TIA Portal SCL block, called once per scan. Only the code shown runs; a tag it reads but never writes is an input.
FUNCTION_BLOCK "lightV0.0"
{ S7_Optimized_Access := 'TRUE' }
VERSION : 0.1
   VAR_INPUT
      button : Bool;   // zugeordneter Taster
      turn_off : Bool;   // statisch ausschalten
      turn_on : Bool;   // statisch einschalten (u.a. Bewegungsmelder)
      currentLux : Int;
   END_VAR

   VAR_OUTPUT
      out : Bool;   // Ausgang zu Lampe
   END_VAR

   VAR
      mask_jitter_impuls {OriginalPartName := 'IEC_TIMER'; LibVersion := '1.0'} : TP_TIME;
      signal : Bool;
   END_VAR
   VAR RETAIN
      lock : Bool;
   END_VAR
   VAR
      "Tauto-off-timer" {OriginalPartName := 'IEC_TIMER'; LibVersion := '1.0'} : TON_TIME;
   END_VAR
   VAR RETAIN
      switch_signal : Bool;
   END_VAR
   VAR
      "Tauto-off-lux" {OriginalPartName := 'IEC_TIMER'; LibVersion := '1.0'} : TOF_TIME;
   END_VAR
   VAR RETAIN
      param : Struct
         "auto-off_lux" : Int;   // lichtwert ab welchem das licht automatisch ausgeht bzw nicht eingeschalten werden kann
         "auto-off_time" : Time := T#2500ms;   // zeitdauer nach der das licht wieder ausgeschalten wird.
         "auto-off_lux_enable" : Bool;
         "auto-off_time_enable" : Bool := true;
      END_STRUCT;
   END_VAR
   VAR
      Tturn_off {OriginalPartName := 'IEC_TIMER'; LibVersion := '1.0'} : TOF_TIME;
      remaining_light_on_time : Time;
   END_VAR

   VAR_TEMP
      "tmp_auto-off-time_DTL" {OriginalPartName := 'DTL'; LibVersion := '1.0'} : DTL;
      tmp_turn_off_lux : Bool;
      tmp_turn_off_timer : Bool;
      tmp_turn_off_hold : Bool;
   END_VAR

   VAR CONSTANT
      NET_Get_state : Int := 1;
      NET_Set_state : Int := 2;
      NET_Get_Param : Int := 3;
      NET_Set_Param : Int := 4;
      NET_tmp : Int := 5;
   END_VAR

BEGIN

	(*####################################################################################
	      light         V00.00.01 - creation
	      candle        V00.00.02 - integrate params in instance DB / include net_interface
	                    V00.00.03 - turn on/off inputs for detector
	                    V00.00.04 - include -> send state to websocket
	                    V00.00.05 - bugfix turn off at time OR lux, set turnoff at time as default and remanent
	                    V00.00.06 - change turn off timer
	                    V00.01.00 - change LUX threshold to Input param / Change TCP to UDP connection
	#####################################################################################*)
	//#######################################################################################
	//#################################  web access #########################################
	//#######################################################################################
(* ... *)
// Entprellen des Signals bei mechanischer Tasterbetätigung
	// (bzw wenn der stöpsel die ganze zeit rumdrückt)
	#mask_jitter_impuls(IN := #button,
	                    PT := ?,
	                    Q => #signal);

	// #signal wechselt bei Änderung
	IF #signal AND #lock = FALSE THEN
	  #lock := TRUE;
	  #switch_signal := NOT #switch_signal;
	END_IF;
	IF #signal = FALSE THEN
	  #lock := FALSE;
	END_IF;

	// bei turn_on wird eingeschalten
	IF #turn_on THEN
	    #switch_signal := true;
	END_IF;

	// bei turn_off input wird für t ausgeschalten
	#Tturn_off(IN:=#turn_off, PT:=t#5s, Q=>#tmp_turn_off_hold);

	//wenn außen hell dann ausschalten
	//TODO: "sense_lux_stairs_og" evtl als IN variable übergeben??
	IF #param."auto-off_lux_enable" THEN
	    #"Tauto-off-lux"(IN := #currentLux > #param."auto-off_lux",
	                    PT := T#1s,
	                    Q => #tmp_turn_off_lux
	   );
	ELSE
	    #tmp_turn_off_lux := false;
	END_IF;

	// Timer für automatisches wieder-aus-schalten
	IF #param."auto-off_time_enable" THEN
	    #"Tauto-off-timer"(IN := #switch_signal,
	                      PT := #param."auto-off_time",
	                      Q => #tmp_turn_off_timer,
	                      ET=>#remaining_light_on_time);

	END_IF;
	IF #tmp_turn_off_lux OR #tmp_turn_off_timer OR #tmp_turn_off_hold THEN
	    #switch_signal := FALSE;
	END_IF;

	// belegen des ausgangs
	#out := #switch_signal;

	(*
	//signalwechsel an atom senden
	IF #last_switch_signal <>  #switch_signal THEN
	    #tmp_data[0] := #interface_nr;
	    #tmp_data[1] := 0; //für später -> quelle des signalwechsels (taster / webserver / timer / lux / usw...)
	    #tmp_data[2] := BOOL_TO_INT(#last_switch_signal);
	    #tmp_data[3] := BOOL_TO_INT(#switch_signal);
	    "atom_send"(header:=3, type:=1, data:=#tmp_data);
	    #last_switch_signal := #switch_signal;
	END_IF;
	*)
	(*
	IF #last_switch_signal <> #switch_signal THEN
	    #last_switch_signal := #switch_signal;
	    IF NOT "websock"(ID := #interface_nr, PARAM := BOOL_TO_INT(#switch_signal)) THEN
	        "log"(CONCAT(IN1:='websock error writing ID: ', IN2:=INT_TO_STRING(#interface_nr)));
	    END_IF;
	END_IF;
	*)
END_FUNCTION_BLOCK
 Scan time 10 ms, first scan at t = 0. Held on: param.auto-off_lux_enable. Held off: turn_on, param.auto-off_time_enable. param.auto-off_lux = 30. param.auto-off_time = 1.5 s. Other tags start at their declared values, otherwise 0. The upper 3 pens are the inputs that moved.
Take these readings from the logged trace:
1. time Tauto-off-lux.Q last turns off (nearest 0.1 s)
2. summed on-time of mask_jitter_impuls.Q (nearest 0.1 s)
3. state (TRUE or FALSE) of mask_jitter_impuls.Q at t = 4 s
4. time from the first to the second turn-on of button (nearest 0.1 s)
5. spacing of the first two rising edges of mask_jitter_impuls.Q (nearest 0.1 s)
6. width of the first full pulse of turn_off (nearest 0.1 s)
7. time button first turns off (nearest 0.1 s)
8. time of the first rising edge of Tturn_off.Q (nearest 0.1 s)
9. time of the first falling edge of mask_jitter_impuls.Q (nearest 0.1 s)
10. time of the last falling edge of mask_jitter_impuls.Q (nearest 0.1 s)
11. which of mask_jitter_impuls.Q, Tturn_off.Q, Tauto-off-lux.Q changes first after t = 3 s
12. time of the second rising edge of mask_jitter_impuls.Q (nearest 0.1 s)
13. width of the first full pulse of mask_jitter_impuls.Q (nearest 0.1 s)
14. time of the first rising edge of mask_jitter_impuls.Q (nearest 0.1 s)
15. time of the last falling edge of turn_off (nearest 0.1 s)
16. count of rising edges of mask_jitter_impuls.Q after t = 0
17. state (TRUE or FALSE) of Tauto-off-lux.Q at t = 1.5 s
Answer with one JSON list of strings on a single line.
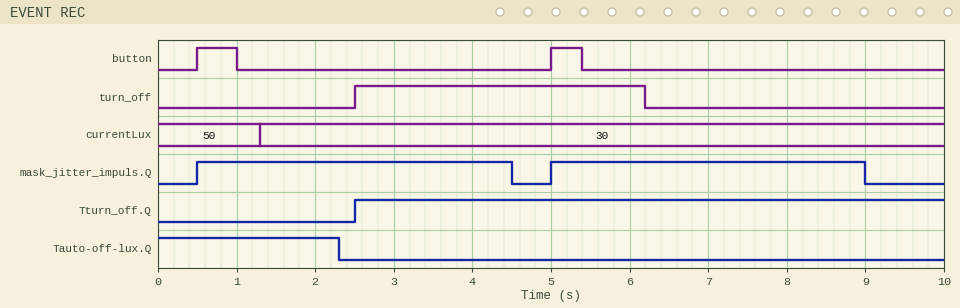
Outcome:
["2.3 s", "8.0 s", "TRUE", "4.5 s", "4.5 s", "3.7 s", "1.0 s", "2.5 s", "4.5 s", "9.0 s", "mask_jitter_impuls.Q", "5.0 s", "4.0 s", "0.5 s", "6.2 s", "2", "TRUE"]
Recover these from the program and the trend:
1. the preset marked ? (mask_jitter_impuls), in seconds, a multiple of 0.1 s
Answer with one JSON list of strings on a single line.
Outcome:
["4.0 s"]
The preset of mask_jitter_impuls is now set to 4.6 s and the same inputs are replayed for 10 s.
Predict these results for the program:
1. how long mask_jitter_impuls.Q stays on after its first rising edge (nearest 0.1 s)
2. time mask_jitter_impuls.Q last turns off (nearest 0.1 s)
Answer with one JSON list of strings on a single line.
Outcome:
["4.6 s", "5.1 s"]
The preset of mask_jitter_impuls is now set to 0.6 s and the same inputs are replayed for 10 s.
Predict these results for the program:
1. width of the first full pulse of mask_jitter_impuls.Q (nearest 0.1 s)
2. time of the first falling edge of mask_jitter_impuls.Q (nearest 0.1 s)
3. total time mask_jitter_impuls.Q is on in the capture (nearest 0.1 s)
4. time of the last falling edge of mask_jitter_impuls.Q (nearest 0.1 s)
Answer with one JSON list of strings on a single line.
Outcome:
["0.6 s", "1.1 s", "1.2 s", "5.6 s"]
